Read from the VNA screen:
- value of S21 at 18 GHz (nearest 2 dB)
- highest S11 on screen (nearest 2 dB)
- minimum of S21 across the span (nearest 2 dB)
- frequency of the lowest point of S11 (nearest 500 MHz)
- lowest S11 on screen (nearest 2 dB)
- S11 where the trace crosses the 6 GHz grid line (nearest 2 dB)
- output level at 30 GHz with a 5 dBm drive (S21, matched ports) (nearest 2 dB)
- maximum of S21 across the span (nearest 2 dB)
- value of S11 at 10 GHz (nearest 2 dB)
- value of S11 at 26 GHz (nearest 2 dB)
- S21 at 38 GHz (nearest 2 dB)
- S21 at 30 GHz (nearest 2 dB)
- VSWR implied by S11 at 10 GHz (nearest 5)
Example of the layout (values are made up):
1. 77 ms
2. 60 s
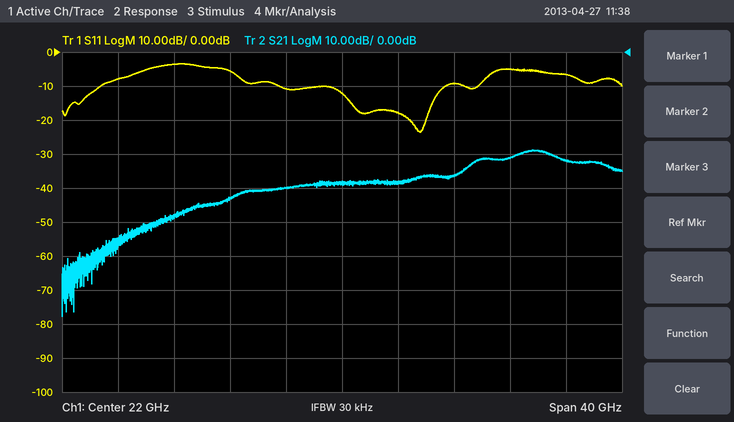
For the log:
1. -40 dB
2. -4 dB
3. -78 dB
4. 27.5 GHz
5. -24 dB
6. -8 dB
7. -32 dBm
8. -28 dB
9. -4 dB
10. -18 dB
11. -32 dB
12. -36 dB
13. 5
